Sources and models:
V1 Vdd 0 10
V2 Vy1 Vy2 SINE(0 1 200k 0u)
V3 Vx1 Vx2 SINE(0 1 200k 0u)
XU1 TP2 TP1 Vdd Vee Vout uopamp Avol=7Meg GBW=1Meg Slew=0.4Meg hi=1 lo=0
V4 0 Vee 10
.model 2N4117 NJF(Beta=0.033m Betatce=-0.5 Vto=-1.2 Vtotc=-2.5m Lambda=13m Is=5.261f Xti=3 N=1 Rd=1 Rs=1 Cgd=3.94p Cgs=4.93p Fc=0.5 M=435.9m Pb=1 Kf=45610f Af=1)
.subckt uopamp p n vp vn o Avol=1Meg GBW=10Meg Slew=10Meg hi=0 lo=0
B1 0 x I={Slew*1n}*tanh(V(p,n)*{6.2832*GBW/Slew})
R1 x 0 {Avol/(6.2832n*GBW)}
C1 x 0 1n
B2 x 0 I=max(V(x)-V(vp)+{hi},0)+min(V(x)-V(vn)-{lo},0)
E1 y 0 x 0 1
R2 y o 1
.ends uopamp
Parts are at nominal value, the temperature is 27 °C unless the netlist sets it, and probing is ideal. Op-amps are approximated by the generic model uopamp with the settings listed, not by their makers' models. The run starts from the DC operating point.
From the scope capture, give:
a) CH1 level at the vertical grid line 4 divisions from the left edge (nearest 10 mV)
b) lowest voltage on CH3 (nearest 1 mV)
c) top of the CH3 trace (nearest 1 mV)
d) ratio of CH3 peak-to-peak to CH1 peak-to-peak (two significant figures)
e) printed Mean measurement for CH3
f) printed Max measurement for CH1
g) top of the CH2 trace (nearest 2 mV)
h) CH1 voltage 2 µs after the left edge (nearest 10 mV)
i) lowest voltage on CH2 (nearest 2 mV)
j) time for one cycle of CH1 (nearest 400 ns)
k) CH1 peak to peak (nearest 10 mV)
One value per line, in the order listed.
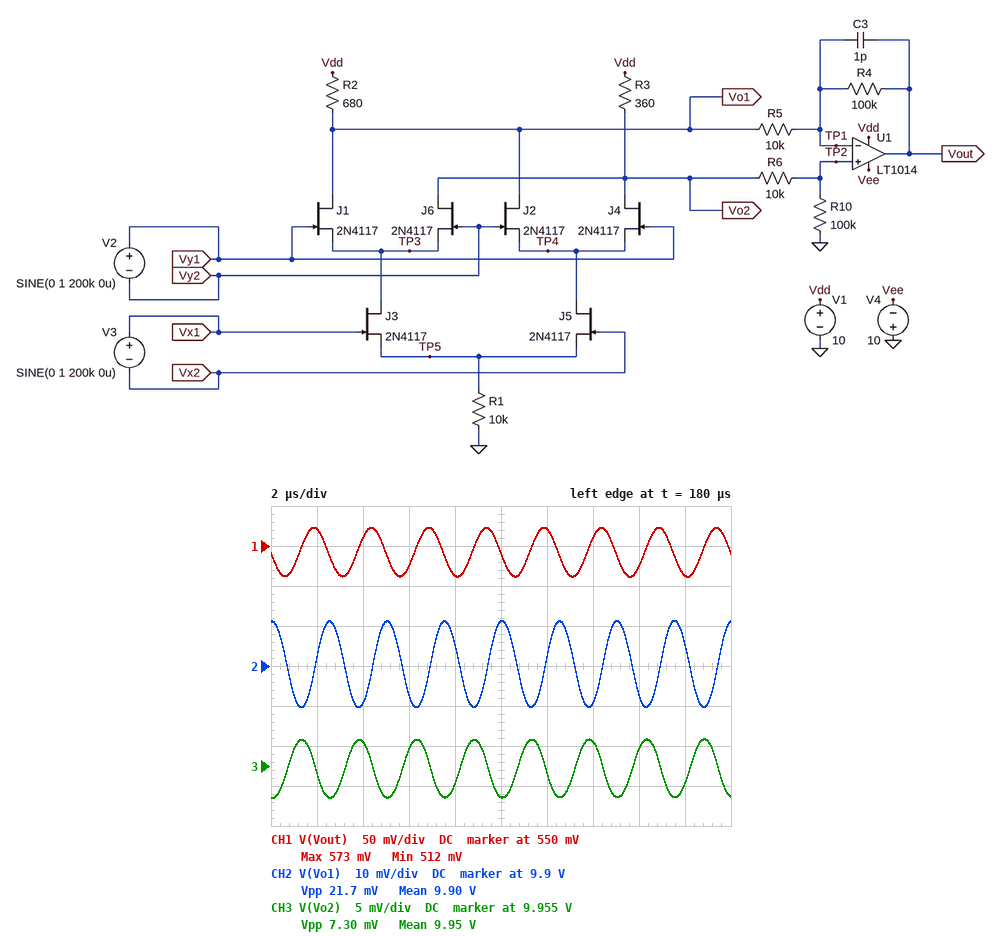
510 mV
9.951 V
9.958 V
0.12
9.95 V
573 mV
9.912 V
570 mV
9.890 V
2.4 µs
60 mV
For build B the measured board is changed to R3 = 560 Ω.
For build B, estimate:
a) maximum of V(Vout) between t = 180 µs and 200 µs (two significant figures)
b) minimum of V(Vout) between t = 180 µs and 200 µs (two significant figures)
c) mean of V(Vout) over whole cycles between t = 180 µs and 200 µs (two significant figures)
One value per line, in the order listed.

340 mV
270 mV
310 mV
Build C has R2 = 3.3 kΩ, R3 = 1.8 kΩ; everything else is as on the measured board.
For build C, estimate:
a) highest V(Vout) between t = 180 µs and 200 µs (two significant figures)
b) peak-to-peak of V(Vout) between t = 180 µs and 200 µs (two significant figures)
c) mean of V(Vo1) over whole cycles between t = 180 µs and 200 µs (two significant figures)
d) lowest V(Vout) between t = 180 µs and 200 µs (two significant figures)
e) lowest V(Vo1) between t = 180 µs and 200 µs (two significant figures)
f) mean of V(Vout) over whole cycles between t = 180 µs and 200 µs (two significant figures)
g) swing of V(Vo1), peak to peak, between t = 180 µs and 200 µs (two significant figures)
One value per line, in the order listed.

2.2 V
250 mV
9.6 V
1.9 V
9.5 V
2.0 V
100 mV
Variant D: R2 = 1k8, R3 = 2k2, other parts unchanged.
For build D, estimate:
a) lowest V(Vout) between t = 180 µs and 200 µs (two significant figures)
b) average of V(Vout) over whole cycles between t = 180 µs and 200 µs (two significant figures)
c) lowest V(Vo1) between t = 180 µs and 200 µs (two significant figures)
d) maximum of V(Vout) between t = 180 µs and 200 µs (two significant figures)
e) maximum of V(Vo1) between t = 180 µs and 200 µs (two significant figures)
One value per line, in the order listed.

-120 mV
-23 mV
9.7 V
76 mV
9.8 V
